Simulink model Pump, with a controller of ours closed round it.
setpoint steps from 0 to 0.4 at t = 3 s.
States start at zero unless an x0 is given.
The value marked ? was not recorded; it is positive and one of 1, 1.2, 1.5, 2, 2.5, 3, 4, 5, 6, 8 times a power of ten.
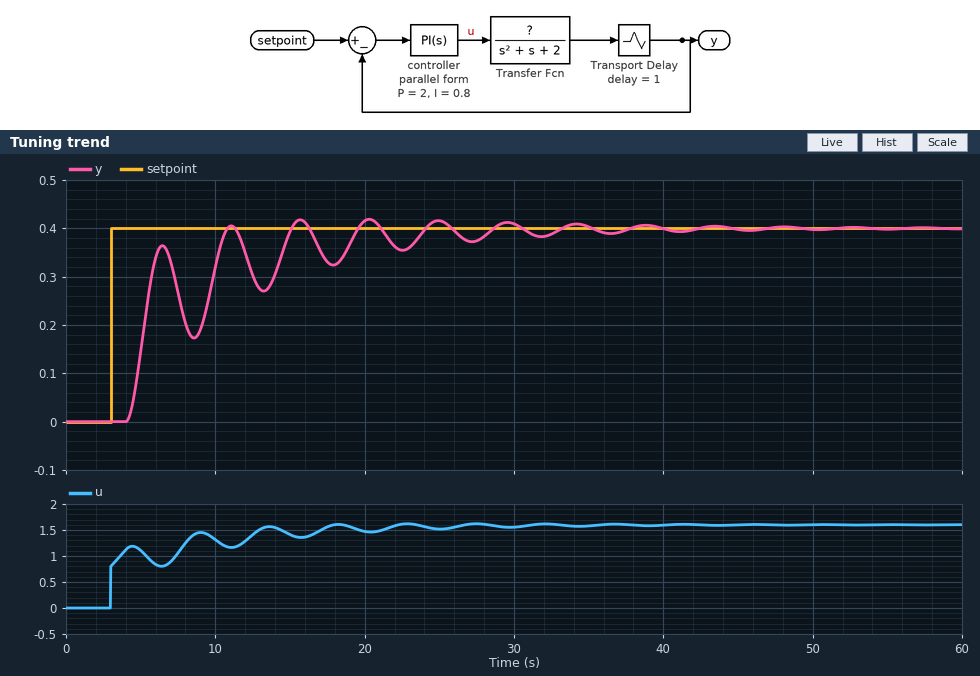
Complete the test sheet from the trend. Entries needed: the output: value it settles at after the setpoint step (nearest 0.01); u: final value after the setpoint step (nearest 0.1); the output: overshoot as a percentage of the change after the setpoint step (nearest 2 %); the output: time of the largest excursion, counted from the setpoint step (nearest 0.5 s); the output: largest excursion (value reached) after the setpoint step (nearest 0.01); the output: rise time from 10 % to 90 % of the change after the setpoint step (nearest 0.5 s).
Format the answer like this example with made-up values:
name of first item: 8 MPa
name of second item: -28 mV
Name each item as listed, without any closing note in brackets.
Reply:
the output: value it settles at after the setpoint step: 0.40
u: final value after the setpoint step: 1.6
the output: overshoot as a percentage of the change after the setpoint step: 4 %
the output: time of the largest excursion, counted from the setpoint step: 17.5 s
the output: largest excursion (value reached) after the setpoint step: 0.42
the output: rise time from 10 % to 90 % of the change after the setpoint step: 2.0 s
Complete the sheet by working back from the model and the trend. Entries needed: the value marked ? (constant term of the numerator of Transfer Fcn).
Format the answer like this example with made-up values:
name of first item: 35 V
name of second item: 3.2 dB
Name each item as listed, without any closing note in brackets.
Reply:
the value marked ?: 0.5
